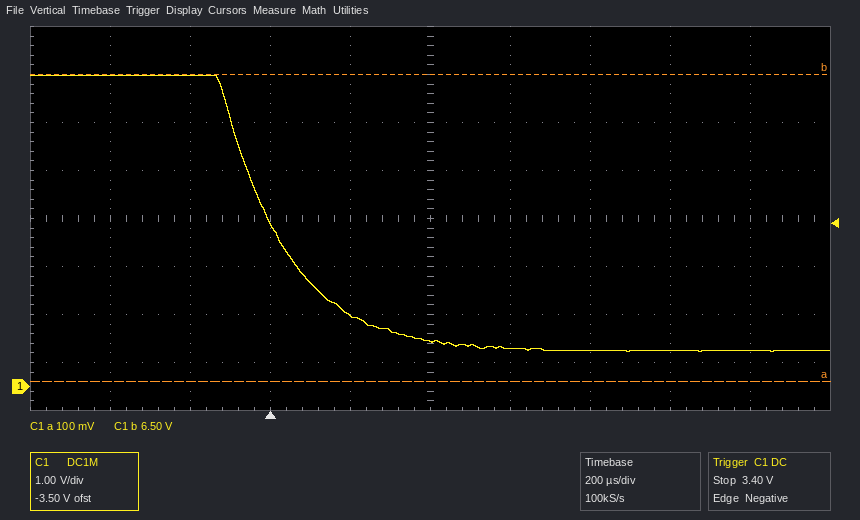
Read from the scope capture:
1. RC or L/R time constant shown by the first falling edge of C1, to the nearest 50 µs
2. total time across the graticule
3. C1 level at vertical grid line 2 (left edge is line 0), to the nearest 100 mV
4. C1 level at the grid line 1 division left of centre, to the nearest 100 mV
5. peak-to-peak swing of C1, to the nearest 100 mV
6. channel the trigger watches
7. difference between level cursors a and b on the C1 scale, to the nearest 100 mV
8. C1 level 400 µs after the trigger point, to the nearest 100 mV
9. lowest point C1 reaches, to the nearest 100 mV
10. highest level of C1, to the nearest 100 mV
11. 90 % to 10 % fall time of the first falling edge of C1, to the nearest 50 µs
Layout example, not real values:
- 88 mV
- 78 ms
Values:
- 150 µs
- 2 ms
- 6.5 V
- 1.5 V
- 5.8 V
- C1
- 6.4 V
- 900 mV
- 700 mV
- 6.5 V
- 350 µs
